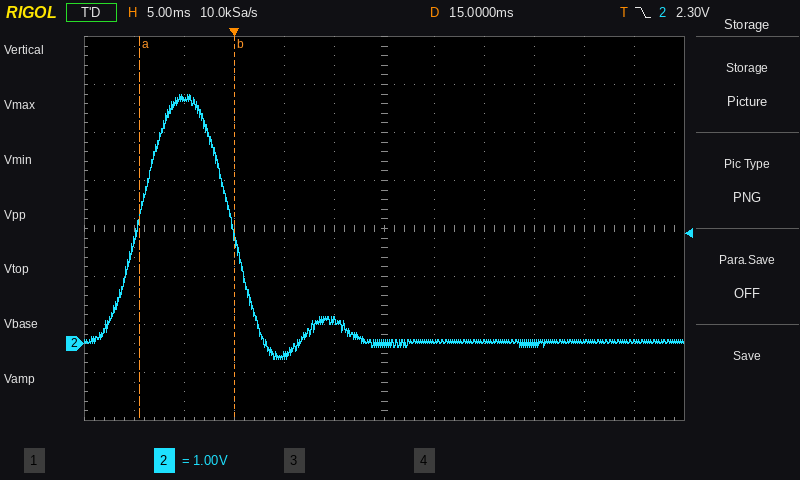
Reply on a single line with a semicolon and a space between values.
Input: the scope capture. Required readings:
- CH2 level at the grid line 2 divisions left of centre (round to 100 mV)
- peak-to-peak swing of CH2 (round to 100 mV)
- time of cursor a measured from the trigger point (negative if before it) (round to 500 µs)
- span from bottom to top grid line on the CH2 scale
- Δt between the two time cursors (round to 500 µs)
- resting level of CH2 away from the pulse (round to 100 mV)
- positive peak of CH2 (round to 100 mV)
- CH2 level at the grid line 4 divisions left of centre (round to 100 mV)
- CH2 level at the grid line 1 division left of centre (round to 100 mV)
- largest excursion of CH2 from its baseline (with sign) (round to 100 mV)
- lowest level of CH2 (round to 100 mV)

-200 mV; 5.5 V; -9.5 ms; 8 V; 9.5 ms; 0.0 V; 5.2 V; 5.1 V; 500 mV; +5.2 V; -300 mV
